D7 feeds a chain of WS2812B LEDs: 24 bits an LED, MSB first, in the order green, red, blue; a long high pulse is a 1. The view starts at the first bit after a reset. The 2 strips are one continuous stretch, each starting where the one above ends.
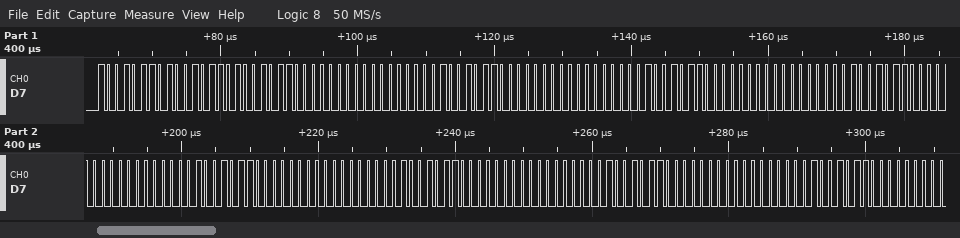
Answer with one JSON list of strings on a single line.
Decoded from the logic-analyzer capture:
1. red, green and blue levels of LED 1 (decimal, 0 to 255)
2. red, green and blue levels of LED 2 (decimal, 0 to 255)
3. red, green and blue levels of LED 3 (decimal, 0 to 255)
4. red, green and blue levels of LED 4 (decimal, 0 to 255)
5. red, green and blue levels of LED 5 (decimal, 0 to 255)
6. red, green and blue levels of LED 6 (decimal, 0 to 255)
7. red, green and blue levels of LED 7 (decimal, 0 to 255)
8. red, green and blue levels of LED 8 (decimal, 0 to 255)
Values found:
["150, 150, 150", "0, 0, 150", "0, 0, 150", "0, 0, 150", "0, 0, 150", "0, 0, 150", "0, 0, 150", "0, 0, 150"]
